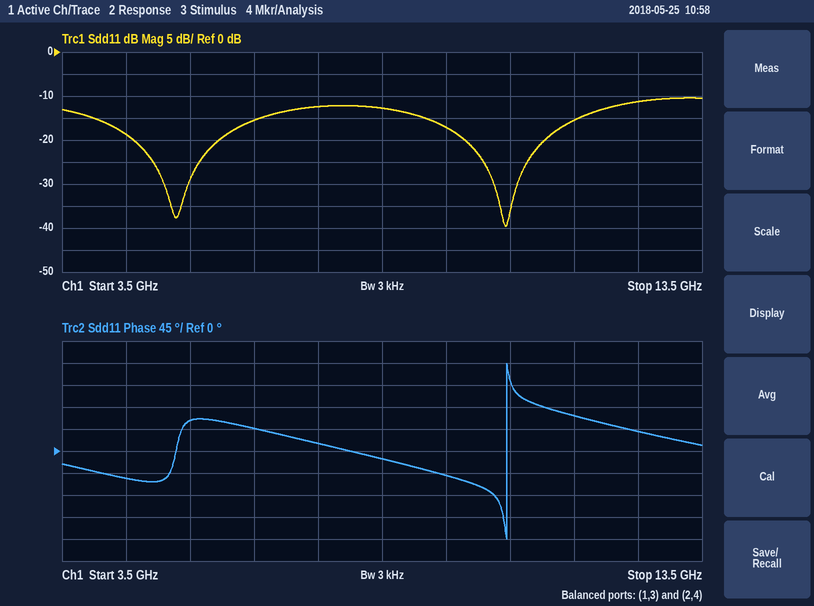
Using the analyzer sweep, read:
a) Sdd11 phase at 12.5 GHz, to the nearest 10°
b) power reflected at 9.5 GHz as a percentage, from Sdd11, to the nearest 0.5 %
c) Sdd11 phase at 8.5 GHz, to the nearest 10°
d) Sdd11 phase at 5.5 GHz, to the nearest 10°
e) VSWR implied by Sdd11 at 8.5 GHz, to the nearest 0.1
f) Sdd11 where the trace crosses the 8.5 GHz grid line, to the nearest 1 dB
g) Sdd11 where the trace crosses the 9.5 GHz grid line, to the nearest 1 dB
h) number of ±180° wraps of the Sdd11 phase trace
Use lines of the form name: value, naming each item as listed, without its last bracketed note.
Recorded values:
Sdd11 phase at 12.5 GHz, to the nearest 10°: 40°
power reflected at 9.5 GHz as a percentage, from Sdd11, to the nearest 0.5 %: 2.0 %
Sdd11 phase at 8.5 GHz, to the nearest 10°: -20°
Sdd11 phase at 5.5 GHz, to the nearest 10°: 60°
VSWR implied by Sdd11 at 8.5 GHz, to the nearest 0.1: 1.6
Sdd11 where the trace crosses the 8.5 GHz grid line, to the nearest 1 dB: -13 dB
Sdd11 where the trace crosses the 9.5 GHz grid line, to the nearest 1 dB: -17 dB
number of ±180° wraps of the Sdd11 phase trace: 1
